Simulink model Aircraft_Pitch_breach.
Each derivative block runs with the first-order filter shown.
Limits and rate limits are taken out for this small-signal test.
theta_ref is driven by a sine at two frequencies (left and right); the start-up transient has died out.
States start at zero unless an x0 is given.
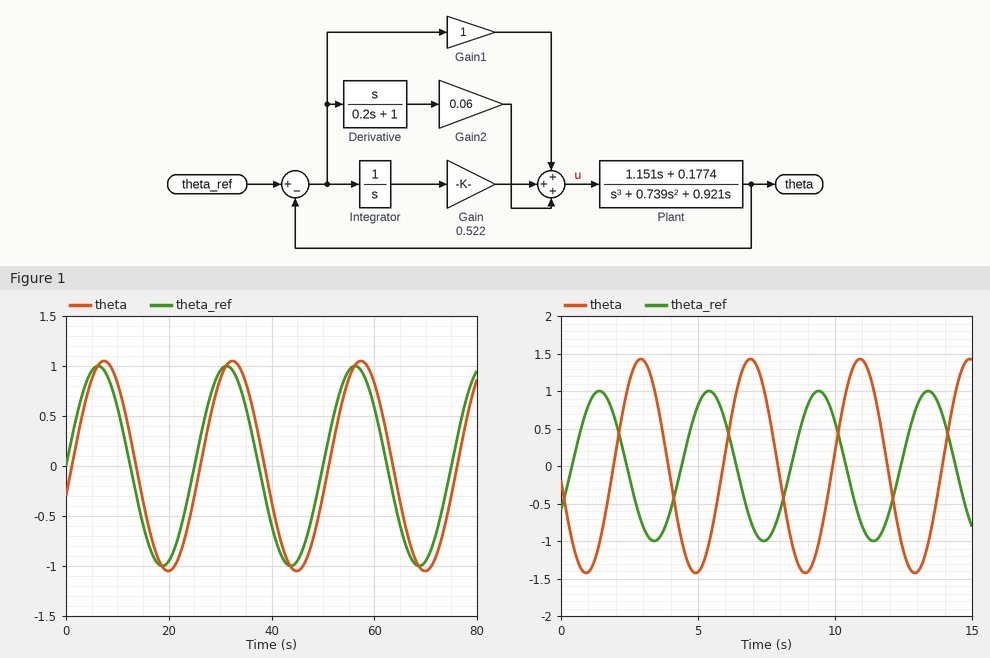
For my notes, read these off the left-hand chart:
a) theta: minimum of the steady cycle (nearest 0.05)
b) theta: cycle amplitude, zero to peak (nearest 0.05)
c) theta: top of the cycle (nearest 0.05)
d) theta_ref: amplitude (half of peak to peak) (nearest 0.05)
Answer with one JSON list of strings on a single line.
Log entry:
["-1.05", "1.05", "1.05", "1.00"]
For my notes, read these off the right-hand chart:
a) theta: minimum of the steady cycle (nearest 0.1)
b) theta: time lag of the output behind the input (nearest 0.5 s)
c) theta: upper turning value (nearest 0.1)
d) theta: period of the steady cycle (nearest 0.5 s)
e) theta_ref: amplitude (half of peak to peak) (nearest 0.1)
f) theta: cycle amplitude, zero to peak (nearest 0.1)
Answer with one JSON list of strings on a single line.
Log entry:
["-1.4", "1.5 s", "1.4", "4.0 s", "1.0", "1.4"]
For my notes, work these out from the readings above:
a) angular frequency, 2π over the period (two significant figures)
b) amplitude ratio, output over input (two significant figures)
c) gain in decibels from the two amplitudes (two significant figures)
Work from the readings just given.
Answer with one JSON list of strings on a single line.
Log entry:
["1.6 rad/s", "1.4", "2.9 dB"]
